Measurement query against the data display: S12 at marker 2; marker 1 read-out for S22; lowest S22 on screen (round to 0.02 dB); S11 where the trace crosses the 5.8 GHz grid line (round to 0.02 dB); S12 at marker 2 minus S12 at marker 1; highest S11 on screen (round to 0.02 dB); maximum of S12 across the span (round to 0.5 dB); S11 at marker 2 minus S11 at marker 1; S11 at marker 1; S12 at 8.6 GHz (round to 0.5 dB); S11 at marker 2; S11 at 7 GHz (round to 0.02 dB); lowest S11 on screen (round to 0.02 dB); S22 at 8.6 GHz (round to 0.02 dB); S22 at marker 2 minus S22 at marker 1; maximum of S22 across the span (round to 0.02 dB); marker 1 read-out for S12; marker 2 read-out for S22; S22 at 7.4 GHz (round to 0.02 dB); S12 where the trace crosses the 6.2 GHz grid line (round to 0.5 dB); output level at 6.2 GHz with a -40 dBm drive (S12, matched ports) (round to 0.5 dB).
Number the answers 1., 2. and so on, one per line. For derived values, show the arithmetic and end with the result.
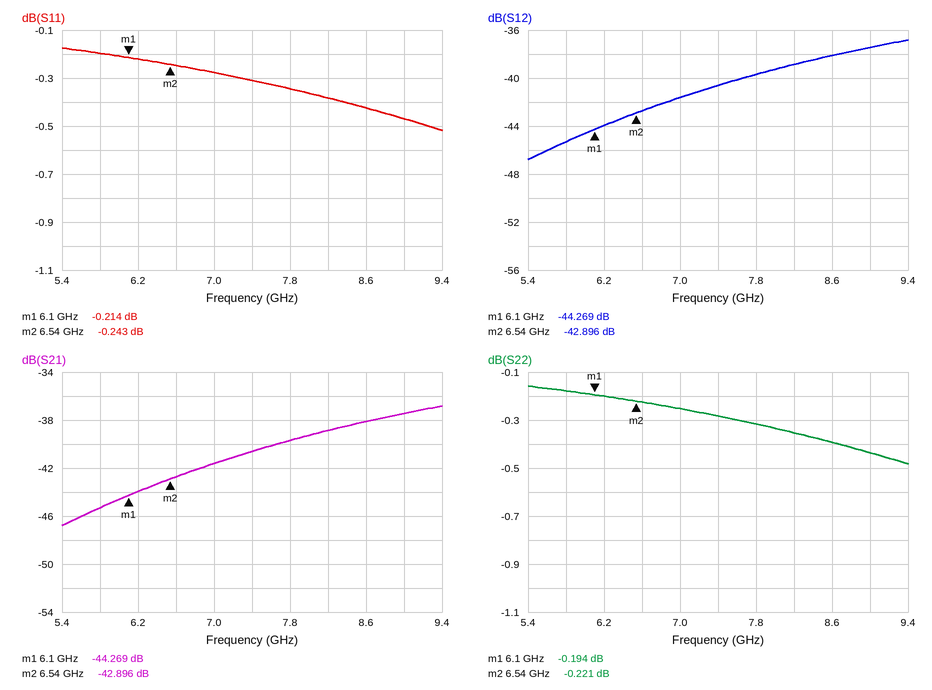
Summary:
1. -42.896 dB
2. -0.194 dB
3. -0.48 dB
4. -0.20 dB
5. -42.896 − (-44.269) = 1.373 dB
6. -0.18 dB
7. -37.0 dB
8. -0.243 − (-0.214) = -0.029 dB
9. -0.214 dB
10. -38.0 dB
11. -0.243 dB
12. -0.28 dB
13. -0.52 dB
14. -0.40 dB
15. -0.221 − (-0.194) = -0.027 dB
16. -0.16 dB
17. -44.269 dB
18. -0.221 dB
19. -0.28 dB
20. -44.0 dB
21. -40 dBm + (-44.0 dB) = -84.0 dBm
